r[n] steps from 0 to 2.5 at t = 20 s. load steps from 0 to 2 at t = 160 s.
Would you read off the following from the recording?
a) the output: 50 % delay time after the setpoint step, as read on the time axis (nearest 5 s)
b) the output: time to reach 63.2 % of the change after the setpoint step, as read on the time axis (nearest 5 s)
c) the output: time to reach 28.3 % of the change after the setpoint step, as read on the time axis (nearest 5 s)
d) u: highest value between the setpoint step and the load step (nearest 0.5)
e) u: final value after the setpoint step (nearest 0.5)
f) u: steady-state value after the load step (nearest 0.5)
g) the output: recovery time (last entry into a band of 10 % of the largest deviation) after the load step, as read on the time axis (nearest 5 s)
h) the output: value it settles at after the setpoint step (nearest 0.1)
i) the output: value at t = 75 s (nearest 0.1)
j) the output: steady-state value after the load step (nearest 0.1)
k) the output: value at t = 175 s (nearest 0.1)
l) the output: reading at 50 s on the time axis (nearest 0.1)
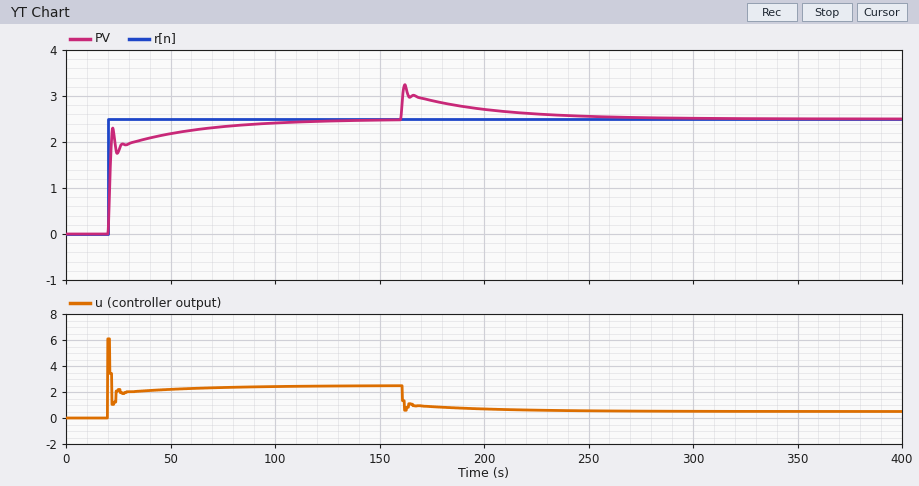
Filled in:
20 s
20 s
20 s
6.0
2.5
0.5
240 s
2.5
2.3
2.5
2.9
2.2
